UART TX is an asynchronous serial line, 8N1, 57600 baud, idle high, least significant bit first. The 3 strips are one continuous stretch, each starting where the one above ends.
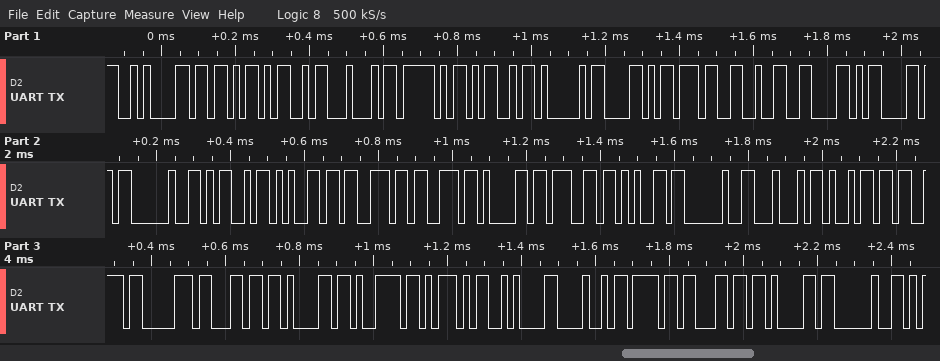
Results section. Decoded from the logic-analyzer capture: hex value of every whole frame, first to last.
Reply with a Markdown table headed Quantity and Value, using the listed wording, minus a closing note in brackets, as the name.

| Quantity | Value |
|---|---|
| hex value of every whole frame, first to last | 0A 5B 4D 44 5F 4D 41 58 37 32 58 58 20 4D 65 73 73 61 67 65 20 44 69 73 70 6C 61 79 5D 0A 48 6F 6C 61 20 |
